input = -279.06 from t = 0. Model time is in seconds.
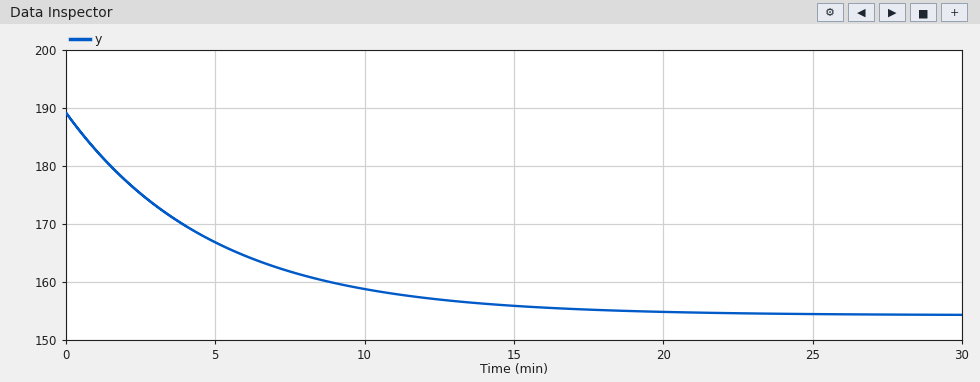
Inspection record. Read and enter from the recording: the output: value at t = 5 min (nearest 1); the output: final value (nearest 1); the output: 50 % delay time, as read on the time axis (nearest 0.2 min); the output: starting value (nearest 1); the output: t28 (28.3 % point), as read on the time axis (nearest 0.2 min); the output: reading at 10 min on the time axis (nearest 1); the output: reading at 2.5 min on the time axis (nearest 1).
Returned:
167
154
3.4 min
189
1.6 min
159
175
